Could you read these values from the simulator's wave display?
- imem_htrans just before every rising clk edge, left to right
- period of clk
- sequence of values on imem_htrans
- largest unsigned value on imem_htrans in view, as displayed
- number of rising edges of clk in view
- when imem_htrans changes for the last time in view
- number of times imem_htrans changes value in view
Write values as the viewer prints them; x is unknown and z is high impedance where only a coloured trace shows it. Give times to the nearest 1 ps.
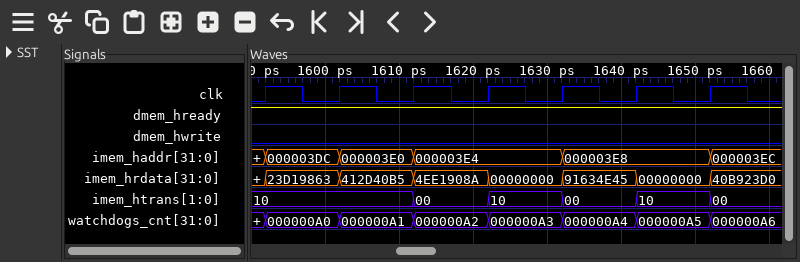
10, 10, 10, 00, 10, 00, 10
10 ps
10, 00, 10, 00, 10, 00
10
7
1652 ps
5
